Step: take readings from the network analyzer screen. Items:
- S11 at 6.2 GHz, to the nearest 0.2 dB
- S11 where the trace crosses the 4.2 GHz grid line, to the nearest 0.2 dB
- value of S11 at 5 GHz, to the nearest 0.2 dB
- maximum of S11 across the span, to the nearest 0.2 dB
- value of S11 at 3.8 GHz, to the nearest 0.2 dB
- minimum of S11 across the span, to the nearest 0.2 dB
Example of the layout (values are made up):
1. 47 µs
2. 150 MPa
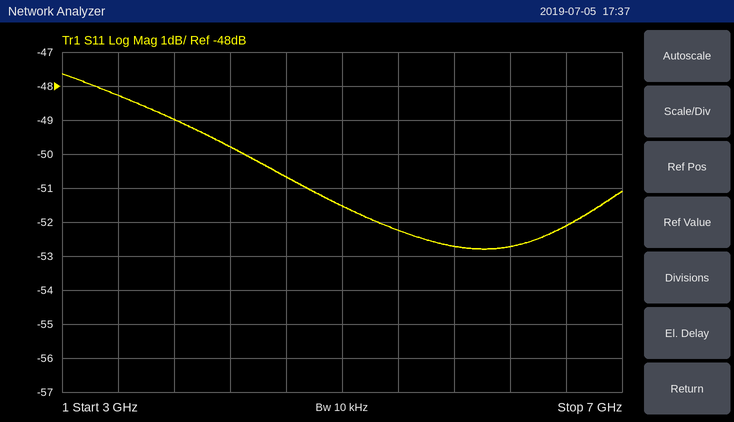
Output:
1. -52.8 dB
2. -49.8 dB
3. -51.6 dB
4. -47.6 dB
5. -49.0 dB
6. -52.8 dB
